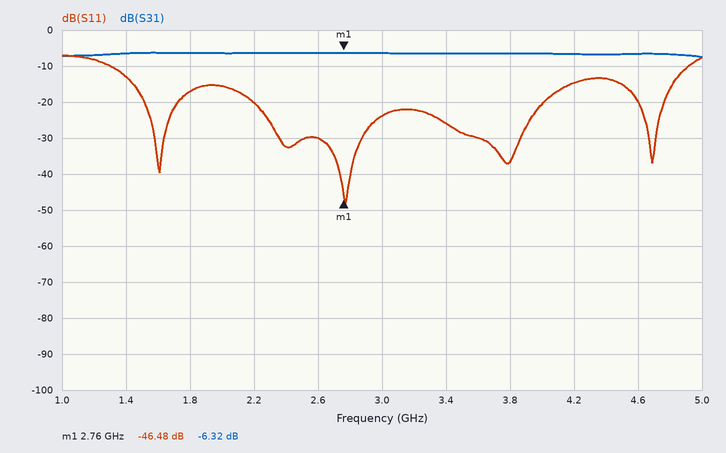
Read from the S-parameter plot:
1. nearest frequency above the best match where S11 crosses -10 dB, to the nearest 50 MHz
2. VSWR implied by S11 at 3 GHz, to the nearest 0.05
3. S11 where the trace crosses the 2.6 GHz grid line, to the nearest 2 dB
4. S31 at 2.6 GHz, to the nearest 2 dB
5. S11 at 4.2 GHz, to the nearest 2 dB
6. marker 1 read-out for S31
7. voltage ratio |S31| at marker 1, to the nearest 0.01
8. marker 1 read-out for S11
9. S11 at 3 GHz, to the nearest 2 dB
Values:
4.90 GHz
1.15
-30 dB
-6 dB
-14 dB
-6.32 dB
0.48
-46.48 dB
-24 dB
